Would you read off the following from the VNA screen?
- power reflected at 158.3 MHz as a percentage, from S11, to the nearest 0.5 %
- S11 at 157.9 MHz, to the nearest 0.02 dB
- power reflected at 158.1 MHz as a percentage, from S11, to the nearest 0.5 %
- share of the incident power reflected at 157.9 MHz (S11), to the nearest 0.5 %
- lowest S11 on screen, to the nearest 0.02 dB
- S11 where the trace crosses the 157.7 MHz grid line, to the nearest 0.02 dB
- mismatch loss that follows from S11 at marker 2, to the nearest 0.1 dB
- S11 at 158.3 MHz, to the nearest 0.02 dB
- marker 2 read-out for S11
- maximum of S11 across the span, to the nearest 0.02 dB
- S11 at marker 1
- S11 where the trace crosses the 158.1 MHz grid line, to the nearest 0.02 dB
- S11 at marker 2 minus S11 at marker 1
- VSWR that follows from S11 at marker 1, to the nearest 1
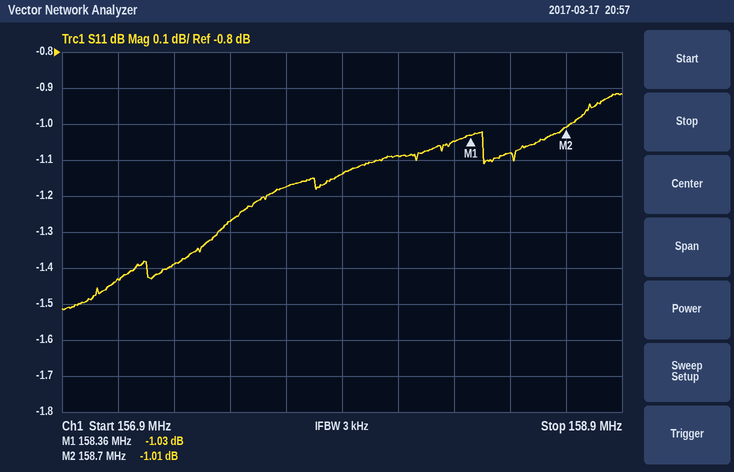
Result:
78.5 %
-1.14 dB
78.0 %
77.0 %
-1.52 dB
-1.18 dB
6.8 dB
-1.04 dB
-1.01 dB
-0.92 dB
-1.03 dB
-1.08 dB
0.02 dB
17
